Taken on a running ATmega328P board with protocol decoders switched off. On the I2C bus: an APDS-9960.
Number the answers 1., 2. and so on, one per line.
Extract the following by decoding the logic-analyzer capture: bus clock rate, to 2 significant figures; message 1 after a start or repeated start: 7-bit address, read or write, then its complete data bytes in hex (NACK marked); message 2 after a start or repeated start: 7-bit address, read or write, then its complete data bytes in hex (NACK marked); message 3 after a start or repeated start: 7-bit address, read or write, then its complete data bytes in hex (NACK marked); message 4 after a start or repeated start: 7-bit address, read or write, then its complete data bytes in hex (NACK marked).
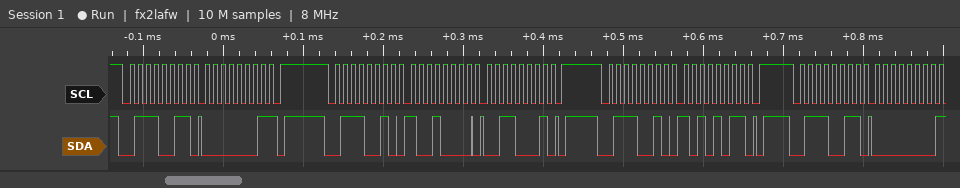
1. 100 kHz
2. 0x39 read: 01 NACK
3. 0x39 write: 90 31
4. 0x39 write: AB
5. 0x39 read: 00 NACK
